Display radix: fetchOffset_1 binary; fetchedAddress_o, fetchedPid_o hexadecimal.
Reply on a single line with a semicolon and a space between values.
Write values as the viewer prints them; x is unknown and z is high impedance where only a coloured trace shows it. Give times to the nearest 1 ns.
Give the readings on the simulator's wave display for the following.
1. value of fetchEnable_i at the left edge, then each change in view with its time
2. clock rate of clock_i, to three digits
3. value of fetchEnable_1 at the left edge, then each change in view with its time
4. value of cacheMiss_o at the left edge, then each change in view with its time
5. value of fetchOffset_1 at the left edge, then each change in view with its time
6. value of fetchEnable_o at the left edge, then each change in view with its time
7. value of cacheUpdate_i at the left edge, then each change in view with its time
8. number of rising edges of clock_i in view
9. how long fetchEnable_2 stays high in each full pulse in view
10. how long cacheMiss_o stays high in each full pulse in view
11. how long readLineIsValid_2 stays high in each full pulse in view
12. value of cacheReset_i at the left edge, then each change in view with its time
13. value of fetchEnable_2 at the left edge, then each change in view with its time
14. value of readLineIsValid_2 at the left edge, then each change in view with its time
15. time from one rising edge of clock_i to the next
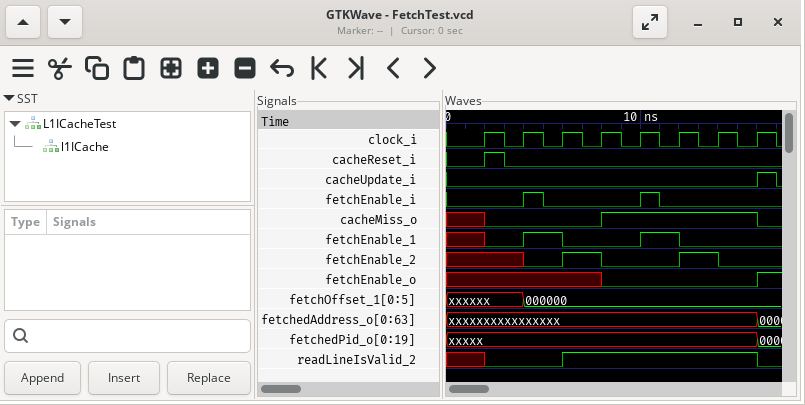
0, 1 at 4 ns, 0 at 5 ns, 1 at 10 ns, 0 at 11 ns; 500 MHz; x, 0 at 2 ns, 1 at 4 ns, 0 at 6 ns, 1 at 10 ns, 0 at 12 ns; x, 0 at 2 ns, 1 at 8 ns, 0 at 16 ns; xxxxxx, 000000 at 4 ns; x, 0 at 8 ns, 1 at 16 ns; 0, 1 at 16 ns, 0 at 17 ns; 8; 2 ns, 2 ns; 8 ns; 10 ns; 0, 1 at 2 ns, 0 at 3 ns; x, 0 at 4 ns, 1 at 6 ns, 0 at 8 ns, 1 at 12 ns, 0 at 14 ns; x, 0 at 2 ns, 1 at 6 ns, 0 at 16 ns; 2 ns
